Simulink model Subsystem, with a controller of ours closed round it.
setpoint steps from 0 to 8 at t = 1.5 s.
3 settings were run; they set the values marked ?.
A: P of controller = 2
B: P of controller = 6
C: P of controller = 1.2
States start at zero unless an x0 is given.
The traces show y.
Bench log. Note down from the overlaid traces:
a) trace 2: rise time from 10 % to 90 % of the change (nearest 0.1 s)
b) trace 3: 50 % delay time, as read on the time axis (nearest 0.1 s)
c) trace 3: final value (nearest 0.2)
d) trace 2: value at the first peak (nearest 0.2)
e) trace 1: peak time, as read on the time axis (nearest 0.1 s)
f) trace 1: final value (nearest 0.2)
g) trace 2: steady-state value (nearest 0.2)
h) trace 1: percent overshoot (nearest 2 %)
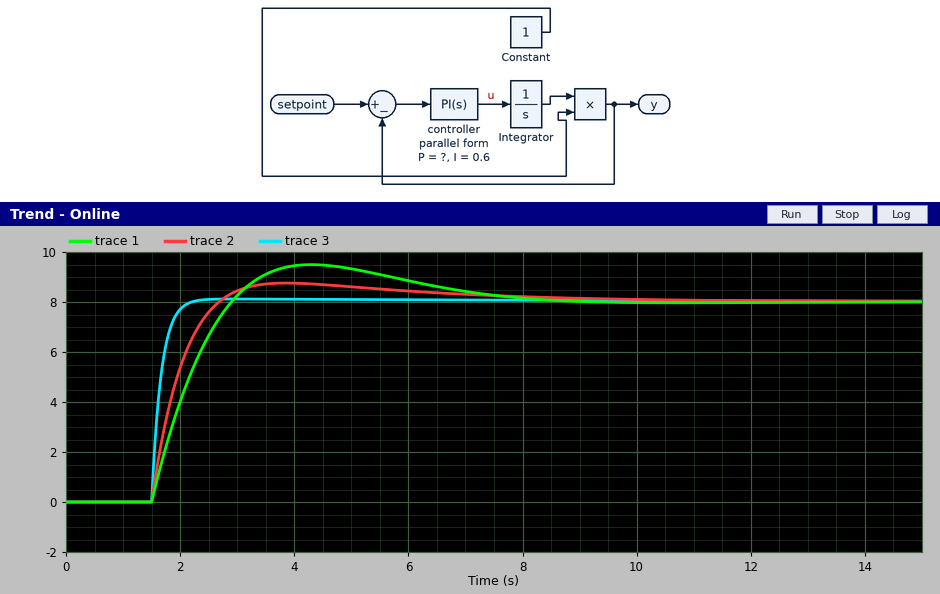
0.8 s
1.6 s
8.0
8.8
4.3 s
8.0
8.0
18 %
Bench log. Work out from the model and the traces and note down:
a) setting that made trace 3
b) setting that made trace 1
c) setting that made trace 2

B
C
A
